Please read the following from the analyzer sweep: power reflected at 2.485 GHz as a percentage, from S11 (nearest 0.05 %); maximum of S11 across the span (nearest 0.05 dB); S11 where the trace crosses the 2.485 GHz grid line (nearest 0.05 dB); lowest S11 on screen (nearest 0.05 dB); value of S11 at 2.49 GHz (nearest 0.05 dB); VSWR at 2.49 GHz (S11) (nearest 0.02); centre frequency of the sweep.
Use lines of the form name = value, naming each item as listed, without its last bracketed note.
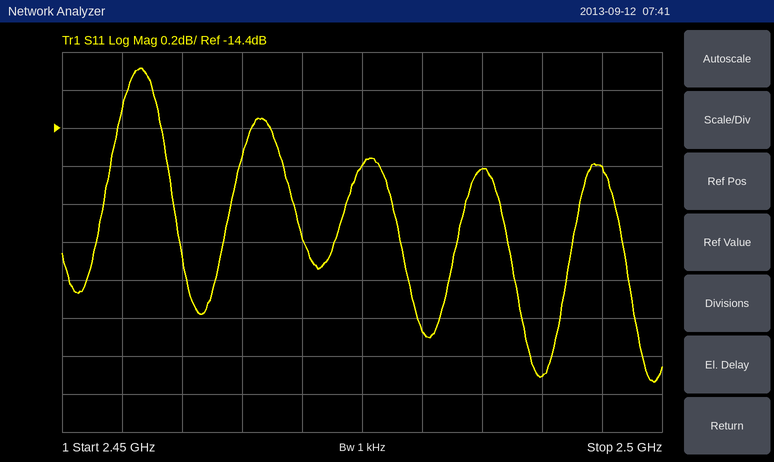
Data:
power reflected at 2.485 GHz as a percentage, from S11 = 3.45 %
maximum of S11 across the span = -14.10 dB
S11 where the trace crosses the 2.485 GHz grid line = -14.60 dB
lowest S11 on screen = -15.75 dB
value of S11 at 2.49 GHz = -15.70 dB
VSWR at 2.49 GHz (S11) = 1.40
centre frequency of the sweep = 2.475 GHz
